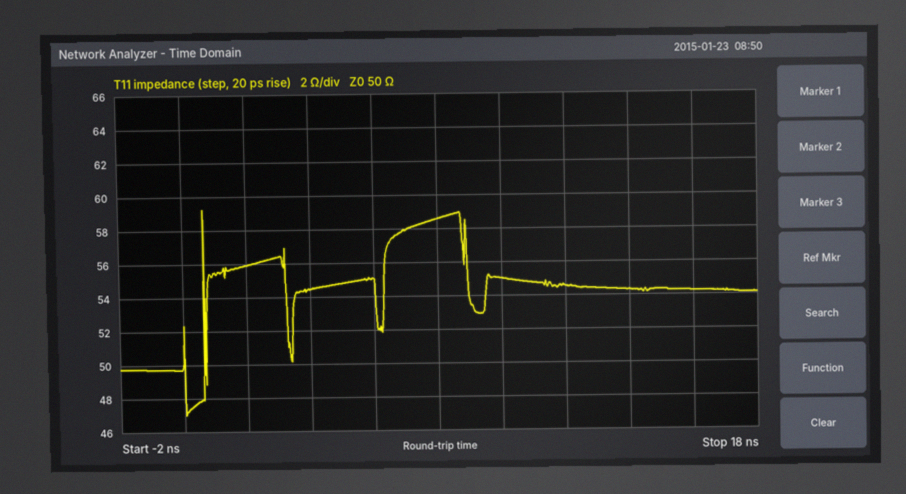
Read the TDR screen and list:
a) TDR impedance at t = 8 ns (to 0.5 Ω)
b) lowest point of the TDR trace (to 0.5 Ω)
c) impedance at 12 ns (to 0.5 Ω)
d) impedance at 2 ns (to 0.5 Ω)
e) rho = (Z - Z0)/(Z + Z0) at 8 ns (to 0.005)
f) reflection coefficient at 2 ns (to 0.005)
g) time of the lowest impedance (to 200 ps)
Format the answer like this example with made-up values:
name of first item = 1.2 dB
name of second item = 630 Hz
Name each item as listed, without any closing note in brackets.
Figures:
TDR impedance at t = 8 ns = 58.5 Ω
lowest point of the TDR trace = 47.0 Ω
impedance at 12 ns = 54.5 Ω
impedance at 2 ns = 56.0 Ω
rho = (Z - Z0)/(Z + Z0) at 8 ns = +0.080
reflection coefficient at 2 ns = +0.055
time of the lowest impedance = 0.0 ns
